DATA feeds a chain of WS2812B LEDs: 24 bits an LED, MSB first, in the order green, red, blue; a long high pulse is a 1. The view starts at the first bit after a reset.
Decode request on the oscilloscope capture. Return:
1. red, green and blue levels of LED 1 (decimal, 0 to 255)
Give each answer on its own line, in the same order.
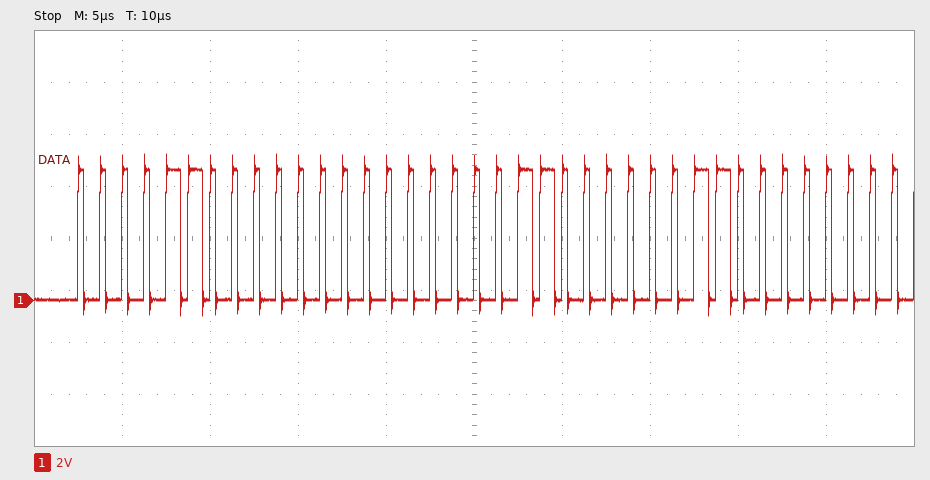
0, 12, 12
